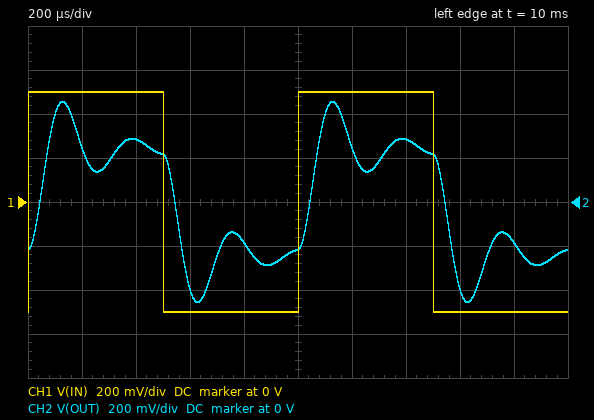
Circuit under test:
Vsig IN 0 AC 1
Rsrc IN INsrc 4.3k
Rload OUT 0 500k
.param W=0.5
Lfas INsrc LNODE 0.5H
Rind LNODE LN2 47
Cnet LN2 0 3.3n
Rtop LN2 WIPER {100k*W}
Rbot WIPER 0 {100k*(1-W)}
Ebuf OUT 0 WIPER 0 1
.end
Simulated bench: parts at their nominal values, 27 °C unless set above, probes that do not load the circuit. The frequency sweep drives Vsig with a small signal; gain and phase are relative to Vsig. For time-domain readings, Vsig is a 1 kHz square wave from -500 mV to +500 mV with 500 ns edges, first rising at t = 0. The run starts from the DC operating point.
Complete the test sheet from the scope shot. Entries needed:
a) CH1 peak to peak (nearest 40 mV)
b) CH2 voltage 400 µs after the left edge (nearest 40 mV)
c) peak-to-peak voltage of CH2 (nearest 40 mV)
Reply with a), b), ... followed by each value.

a) 1.00 V
b) 280 mV
c) 920 mV
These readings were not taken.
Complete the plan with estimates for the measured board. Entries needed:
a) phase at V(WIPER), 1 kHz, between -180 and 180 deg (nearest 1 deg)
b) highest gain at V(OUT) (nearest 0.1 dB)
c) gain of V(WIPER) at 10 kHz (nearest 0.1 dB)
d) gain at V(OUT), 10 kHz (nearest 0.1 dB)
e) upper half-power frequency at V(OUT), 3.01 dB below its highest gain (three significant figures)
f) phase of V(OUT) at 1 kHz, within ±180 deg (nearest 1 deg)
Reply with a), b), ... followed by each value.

a) -7 deg
b) 0.5 dB
c) -21.0 dB
d) -21.0 dB
e) 4.64 kHz
f) -7 deg
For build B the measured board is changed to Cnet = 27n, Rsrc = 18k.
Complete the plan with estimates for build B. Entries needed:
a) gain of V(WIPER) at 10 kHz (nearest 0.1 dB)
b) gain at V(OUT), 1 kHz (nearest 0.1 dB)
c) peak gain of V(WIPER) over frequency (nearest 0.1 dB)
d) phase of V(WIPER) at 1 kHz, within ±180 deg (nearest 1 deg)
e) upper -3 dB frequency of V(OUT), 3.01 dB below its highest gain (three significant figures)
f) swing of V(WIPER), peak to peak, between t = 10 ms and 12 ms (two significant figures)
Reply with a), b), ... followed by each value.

a) -41.7 dB
b) -16.0 dB
c) -7.5 dB
d) -78 deg
e) 408 Hz
f) 230 mV
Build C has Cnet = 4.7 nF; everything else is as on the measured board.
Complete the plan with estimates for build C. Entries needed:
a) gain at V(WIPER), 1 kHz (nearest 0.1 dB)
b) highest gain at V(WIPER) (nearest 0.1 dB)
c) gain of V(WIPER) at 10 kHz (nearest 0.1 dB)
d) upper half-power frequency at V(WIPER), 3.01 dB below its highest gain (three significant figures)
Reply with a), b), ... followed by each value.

a) -5.7 dB
b) -0.3 dB
c) -24.5 dB
d) 3.92 kHz
